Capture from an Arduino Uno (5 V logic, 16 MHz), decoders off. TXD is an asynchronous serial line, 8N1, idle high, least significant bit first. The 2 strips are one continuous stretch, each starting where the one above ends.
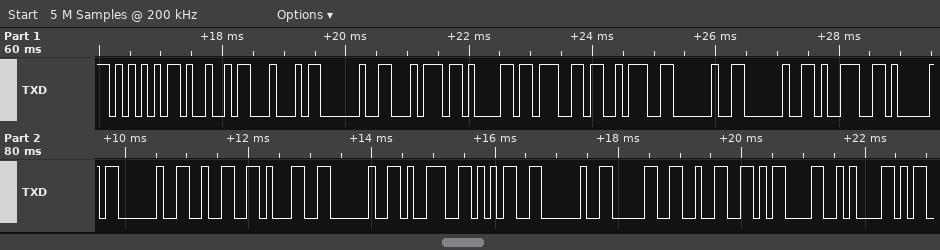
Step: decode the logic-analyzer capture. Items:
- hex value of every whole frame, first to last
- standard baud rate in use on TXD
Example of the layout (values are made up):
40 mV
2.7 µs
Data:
55 49 44 20 74 61 67 3A 20 20 39 41 20 32 31 20 39 35 20 30 32 0D 0A
9600 baud
